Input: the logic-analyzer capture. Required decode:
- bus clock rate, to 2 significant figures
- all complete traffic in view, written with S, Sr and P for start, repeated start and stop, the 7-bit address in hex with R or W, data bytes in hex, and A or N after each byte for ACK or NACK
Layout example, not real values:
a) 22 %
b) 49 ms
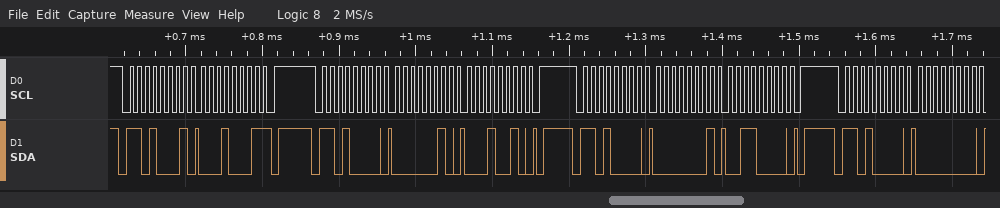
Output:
a) 100 kHz
b) S 68R A 11 N P S 68W A 02 A 12 A P S 68W A 01 A 30 A P S 68W A 00 A
